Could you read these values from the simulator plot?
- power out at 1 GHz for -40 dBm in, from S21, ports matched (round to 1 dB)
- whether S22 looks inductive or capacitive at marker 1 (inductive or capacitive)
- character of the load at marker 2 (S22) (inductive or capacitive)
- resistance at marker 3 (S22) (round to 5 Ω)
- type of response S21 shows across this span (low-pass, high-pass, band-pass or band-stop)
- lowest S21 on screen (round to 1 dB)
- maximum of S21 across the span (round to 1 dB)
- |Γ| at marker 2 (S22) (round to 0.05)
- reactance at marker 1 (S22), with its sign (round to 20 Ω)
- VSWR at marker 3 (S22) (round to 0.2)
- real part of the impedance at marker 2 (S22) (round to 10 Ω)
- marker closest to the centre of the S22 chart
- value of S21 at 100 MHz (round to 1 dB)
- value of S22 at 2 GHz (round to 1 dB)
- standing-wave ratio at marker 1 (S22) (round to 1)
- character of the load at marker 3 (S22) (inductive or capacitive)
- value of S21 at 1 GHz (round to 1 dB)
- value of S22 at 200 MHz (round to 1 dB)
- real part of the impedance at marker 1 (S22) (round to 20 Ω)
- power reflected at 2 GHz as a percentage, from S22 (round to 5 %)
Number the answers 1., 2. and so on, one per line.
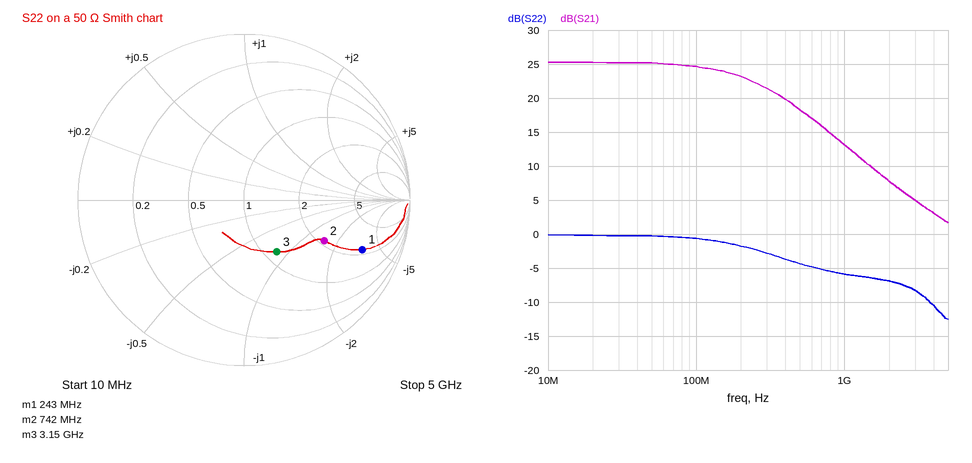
1. -27 dBm
2. capacitive
3. capacitive
4. 60 Ω
5. low-pass
6. 2 dB
7. 25 dB
8. 0.55
9. -180 Ω
10. 2.2
11. 110 Ω
12. marker 3
13. 25 dB
14. -7 dB
15. 8
16. capacitive
17. 13 dB
18. -2 dB
19. 120 Ω
20. 20 %
